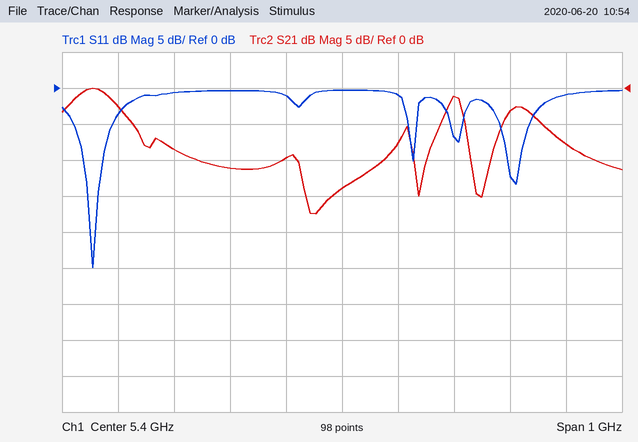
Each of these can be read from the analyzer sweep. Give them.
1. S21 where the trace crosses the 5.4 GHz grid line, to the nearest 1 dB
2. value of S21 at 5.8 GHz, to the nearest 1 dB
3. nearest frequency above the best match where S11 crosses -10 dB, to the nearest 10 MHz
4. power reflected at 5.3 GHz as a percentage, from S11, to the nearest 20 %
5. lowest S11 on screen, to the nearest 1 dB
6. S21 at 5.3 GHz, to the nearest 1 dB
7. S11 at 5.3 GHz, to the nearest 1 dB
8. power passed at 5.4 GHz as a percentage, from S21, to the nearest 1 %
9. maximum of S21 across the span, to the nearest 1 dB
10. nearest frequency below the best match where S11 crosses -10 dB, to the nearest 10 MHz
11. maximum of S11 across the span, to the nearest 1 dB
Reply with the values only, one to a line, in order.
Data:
-14 dB
-8 dB
4.97 GHz
80 %
-25 dB
-10 dB
-1 dB
4 %
0 dB
4.94 GHz
0 dB
